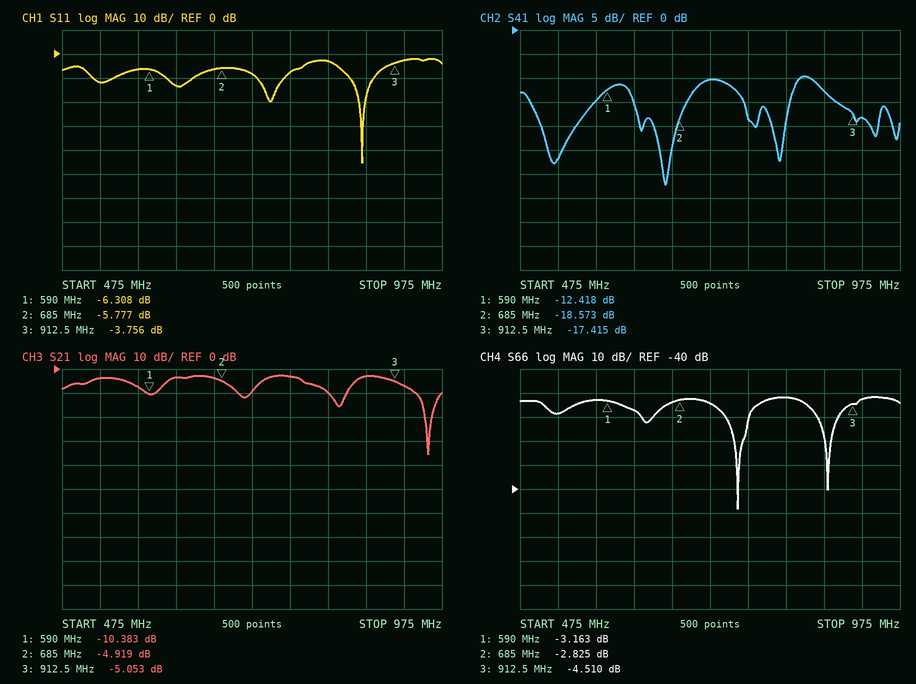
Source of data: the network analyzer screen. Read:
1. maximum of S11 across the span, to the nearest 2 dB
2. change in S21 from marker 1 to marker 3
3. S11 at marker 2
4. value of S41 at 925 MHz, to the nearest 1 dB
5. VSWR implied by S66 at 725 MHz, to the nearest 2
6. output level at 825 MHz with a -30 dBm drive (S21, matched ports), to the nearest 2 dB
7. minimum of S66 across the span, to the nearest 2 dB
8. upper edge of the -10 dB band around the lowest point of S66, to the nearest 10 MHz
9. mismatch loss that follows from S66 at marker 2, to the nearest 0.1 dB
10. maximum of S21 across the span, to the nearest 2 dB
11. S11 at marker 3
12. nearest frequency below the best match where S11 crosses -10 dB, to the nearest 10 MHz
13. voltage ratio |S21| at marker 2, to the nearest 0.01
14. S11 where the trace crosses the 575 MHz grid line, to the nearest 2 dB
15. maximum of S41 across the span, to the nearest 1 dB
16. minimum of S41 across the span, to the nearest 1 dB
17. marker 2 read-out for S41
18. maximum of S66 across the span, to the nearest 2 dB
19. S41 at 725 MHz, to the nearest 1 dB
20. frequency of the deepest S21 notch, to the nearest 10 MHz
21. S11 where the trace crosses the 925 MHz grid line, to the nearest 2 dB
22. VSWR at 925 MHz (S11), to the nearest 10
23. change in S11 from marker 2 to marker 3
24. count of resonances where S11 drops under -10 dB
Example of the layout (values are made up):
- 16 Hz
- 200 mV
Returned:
- -2 dB
- 5.330 dB
- -5.777 dB
- -18 dB
- 4
- -40 dBm
- -48 dB
- 780 MHz
- 3.2 dB
- -2 dB
- -3.756 dB
- 850 MHz
- 0.57
- -6 dB
- -10 dB
- -32 dB
- -18.573 dB
- -2 dB
- -10 dB
- 960 MHz
- -2 dB
- 10
- 2.021 dB
- 4
